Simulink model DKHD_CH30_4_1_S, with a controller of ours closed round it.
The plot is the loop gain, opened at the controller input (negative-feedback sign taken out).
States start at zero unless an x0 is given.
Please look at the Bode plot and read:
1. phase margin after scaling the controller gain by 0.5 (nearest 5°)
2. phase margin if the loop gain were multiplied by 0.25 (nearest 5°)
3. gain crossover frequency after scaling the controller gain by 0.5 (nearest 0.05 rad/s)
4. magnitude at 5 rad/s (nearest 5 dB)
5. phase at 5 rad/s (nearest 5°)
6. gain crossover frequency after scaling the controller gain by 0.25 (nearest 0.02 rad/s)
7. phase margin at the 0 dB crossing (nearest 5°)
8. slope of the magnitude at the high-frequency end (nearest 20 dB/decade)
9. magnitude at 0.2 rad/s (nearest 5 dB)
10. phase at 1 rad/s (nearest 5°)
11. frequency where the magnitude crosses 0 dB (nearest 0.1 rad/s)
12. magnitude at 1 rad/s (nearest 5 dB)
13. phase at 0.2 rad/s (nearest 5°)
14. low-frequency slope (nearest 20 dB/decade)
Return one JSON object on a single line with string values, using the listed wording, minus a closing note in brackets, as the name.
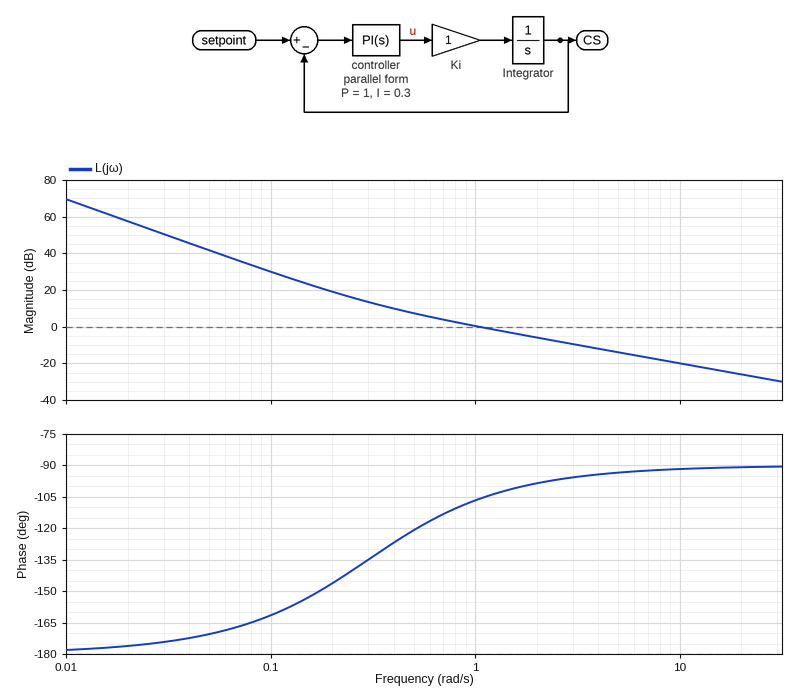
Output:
{"phase margin after scaling the controller gain by 0.5": "60°", "phase margin if the loop gain were multiplied by 0.25": "50°", "gain crossover frequency after scaling the controller gain by 0.5": "0.55 rad/s", "magnitude at 5 rad/s": "-15 dB", "phase at 5 rad/s": "-95°", "gain crossover frequency after scaling the controller gain by 0.25": "0.34 rad/s", "phase margin at the 0 dB crossing": "75°", "slope of the magnitude at the high-frequency end": "-20 dB/decade", "magnitude at 0.2 rad/s": "20 dB", "phase at 1 rad/s": "-105°", "frequency where the magnitude crosses 0 dB": "1.0 rad/s", "magnitude at 1 rad/s": "0 dB", "phase at 0.2 rad/s": "-145°", "low-frequency slope": "-40 dB/decade"}
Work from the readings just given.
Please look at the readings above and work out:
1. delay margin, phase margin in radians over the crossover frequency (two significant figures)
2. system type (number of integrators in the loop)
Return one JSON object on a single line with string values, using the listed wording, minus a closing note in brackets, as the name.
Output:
{"delay margin, phase margin in radians over the crossover frequency": "1.3 s", "system type": "2"}
